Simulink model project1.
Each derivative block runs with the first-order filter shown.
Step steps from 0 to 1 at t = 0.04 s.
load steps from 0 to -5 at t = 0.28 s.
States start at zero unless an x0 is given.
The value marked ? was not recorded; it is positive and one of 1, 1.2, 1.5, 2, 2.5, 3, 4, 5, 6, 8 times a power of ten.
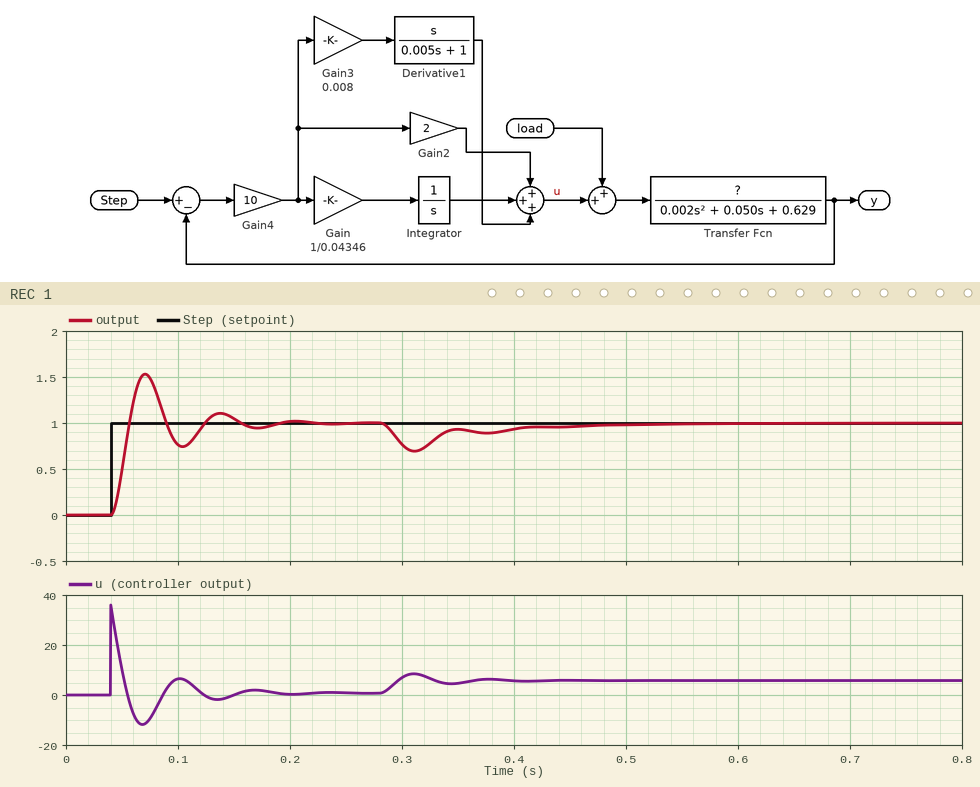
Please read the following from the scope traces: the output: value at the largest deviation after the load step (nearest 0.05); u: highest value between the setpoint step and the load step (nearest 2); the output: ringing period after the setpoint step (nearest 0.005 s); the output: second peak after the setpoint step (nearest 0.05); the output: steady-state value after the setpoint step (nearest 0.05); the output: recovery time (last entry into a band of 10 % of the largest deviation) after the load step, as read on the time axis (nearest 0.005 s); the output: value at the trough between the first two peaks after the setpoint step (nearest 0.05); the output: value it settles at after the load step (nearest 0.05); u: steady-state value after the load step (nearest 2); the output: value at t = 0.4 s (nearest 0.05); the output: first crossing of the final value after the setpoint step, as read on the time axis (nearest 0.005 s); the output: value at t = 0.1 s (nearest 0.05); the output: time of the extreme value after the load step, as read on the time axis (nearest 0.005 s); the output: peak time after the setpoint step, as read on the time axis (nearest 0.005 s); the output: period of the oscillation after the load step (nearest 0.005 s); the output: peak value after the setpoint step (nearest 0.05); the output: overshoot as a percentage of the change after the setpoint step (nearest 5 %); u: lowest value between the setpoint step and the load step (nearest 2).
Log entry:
0.70
36
0.065 s
1.10
1.00
0.465 s
0.75
1.00
6
0.95
0.055 s
0.75
0.310 s
0.070 s
0.065 s
1.55
55 %
-12
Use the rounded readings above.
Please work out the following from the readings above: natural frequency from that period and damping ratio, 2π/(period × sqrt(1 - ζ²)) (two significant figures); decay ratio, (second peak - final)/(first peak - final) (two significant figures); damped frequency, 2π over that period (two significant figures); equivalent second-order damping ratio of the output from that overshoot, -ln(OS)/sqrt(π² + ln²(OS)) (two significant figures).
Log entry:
98 rad/s
0.18
97 rad/s
0.19
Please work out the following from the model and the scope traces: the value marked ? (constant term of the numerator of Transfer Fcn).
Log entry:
0.8
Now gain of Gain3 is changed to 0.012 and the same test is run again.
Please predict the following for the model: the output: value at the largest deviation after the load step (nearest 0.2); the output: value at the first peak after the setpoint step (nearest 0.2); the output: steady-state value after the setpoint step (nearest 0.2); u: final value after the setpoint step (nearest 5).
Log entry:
0.8
1.4
1.0
0
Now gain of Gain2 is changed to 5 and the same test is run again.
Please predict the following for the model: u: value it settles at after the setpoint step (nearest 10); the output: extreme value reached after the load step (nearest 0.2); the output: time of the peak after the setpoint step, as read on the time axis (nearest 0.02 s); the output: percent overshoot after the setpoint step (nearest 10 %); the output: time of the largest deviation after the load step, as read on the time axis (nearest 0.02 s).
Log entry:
0
0.8
0.06 s
70 %
0.30 s
